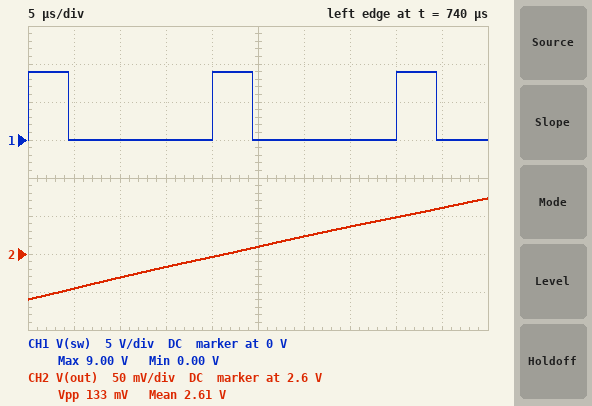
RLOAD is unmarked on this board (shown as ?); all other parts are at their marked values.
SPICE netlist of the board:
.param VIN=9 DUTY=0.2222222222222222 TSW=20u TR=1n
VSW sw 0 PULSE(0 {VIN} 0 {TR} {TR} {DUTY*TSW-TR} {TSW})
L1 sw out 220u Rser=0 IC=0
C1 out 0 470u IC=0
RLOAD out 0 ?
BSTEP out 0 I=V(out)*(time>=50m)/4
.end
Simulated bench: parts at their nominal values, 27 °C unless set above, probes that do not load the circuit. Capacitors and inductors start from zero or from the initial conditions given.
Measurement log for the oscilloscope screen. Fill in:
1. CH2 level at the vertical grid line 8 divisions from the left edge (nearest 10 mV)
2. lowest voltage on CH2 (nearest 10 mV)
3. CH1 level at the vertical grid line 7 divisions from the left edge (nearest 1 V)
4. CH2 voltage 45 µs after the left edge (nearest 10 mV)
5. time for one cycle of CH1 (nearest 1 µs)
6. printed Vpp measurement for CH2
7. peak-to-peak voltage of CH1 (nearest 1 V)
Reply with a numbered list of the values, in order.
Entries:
1. 2.65 V
2. 2.54 V
3. 0 V
4. 2.66 V
5. 20 µs
6. 133 mV
7. 9 V
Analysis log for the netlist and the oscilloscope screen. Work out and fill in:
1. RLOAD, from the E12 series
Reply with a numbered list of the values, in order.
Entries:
1. 1.5 Ω
